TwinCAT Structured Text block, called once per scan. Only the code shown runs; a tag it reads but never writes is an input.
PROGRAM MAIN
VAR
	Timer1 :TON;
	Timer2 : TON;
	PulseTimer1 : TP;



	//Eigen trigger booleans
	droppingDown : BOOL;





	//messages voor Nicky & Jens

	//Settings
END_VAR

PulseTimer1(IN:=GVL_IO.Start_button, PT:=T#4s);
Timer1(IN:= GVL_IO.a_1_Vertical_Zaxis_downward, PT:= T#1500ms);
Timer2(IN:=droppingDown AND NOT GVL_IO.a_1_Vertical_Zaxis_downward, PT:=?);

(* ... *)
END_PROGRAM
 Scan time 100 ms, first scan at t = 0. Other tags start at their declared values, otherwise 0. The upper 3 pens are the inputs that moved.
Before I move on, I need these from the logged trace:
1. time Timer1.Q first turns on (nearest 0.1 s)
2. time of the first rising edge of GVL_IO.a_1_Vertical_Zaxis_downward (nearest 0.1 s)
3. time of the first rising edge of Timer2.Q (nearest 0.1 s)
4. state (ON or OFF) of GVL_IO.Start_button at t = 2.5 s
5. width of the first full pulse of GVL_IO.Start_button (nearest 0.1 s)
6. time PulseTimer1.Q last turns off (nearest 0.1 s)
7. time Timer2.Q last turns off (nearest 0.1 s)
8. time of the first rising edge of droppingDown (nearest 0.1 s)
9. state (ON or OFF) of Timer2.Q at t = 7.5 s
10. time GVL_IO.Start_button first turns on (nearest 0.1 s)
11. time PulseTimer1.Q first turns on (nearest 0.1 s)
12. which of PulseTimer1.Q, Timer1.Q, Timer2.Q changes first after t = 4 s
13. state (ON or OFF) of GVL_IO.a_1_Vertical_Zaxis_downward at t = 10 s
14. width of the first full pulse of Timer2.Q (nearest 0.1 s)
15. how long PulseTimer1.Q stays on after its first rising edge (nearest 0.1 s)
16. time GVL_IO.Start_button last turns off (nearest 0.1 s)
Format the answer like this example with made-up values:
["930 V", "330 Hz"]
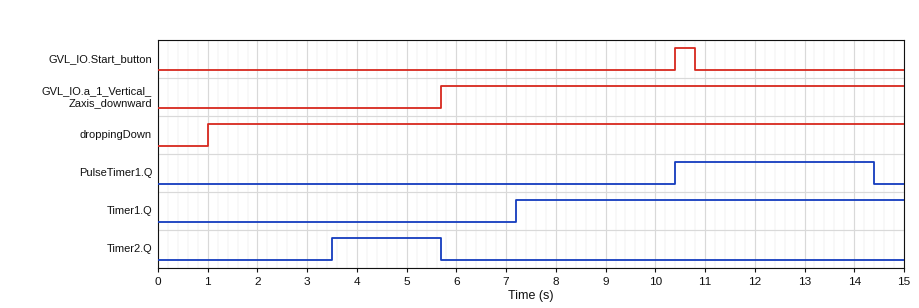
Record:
["7.2 s", "5.7 s", "3.5 s", "OFF", "0.4 s", "14.4 s", "5.7 s", "1.0 s", "OFF", "10.4 s", "10.4 s", "Timer2.Q", "ON", "2.2 s", "4.0 s", "10.8 s"]
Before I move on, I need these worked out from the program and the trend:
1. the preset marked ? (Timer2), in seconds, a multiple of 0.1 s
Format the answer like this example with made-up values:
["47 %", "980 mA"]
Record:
["2.5 s"]
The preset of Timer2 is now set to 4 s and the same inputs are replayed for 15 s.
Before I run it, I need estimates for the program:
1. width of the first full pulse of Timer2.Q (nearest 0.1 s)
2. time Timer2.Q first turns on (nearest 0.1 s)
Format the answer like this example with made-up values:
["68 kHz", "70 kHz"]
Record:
["0.7 s", "5.0 s"]
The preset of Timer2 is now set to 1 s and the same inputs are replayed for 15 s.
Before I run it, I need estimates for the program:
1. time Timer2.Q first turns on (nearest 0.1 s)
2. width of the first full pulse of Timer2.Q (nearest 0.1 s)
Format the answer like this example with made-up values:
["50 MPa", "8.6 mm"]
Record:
["2.0 s", "3.7 s"]
